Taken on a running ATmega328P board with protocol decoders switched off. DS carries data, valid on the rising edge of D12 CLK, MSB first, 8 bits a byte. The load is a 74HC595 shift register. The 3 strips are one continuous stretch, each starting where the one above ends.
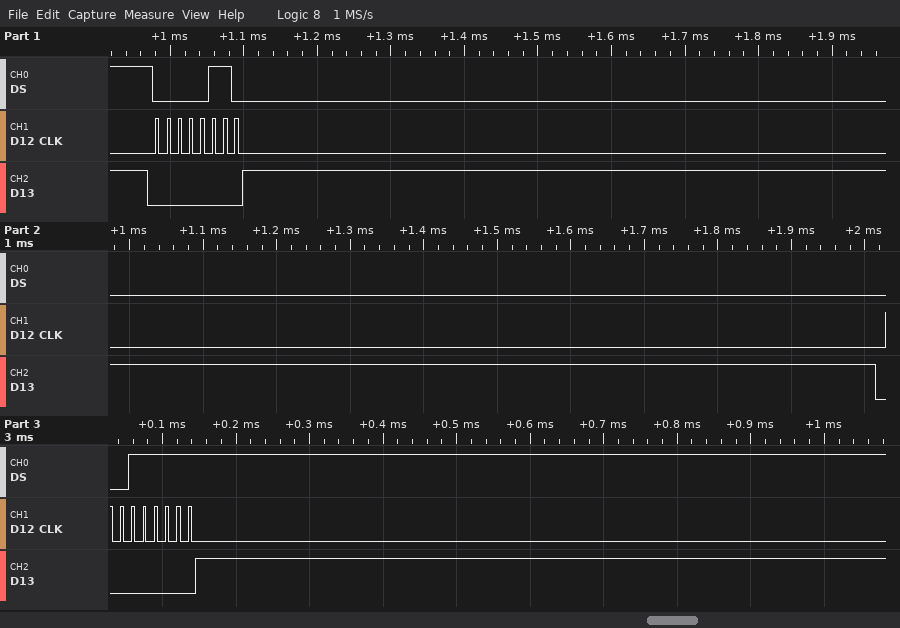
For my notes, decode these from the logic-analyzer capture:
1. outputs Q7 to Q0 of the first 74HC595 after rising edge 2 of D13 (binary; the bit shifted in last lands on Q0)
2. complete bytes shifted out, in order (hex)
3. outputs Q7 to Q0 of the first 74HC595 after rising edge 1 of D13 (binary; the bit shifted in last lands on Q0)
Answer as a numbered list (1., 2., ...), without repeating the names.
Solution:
1. 00111111
2. 06 3F
3. 00000110
